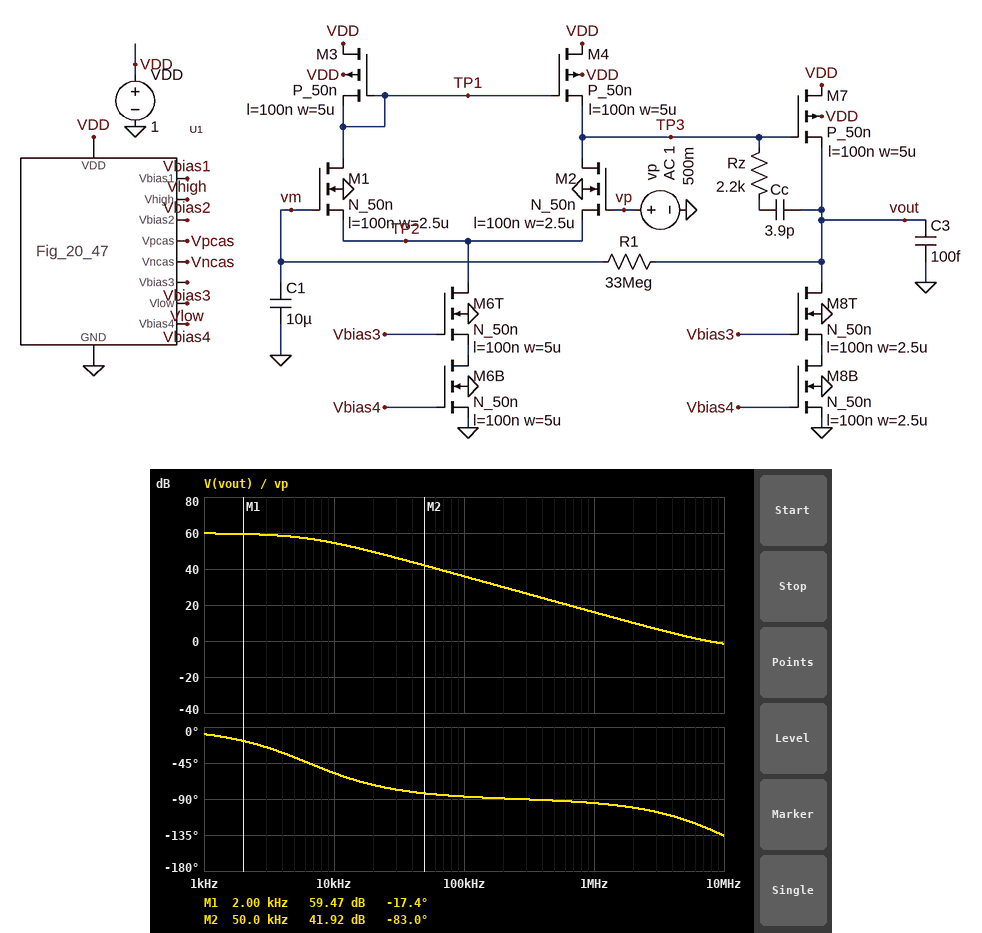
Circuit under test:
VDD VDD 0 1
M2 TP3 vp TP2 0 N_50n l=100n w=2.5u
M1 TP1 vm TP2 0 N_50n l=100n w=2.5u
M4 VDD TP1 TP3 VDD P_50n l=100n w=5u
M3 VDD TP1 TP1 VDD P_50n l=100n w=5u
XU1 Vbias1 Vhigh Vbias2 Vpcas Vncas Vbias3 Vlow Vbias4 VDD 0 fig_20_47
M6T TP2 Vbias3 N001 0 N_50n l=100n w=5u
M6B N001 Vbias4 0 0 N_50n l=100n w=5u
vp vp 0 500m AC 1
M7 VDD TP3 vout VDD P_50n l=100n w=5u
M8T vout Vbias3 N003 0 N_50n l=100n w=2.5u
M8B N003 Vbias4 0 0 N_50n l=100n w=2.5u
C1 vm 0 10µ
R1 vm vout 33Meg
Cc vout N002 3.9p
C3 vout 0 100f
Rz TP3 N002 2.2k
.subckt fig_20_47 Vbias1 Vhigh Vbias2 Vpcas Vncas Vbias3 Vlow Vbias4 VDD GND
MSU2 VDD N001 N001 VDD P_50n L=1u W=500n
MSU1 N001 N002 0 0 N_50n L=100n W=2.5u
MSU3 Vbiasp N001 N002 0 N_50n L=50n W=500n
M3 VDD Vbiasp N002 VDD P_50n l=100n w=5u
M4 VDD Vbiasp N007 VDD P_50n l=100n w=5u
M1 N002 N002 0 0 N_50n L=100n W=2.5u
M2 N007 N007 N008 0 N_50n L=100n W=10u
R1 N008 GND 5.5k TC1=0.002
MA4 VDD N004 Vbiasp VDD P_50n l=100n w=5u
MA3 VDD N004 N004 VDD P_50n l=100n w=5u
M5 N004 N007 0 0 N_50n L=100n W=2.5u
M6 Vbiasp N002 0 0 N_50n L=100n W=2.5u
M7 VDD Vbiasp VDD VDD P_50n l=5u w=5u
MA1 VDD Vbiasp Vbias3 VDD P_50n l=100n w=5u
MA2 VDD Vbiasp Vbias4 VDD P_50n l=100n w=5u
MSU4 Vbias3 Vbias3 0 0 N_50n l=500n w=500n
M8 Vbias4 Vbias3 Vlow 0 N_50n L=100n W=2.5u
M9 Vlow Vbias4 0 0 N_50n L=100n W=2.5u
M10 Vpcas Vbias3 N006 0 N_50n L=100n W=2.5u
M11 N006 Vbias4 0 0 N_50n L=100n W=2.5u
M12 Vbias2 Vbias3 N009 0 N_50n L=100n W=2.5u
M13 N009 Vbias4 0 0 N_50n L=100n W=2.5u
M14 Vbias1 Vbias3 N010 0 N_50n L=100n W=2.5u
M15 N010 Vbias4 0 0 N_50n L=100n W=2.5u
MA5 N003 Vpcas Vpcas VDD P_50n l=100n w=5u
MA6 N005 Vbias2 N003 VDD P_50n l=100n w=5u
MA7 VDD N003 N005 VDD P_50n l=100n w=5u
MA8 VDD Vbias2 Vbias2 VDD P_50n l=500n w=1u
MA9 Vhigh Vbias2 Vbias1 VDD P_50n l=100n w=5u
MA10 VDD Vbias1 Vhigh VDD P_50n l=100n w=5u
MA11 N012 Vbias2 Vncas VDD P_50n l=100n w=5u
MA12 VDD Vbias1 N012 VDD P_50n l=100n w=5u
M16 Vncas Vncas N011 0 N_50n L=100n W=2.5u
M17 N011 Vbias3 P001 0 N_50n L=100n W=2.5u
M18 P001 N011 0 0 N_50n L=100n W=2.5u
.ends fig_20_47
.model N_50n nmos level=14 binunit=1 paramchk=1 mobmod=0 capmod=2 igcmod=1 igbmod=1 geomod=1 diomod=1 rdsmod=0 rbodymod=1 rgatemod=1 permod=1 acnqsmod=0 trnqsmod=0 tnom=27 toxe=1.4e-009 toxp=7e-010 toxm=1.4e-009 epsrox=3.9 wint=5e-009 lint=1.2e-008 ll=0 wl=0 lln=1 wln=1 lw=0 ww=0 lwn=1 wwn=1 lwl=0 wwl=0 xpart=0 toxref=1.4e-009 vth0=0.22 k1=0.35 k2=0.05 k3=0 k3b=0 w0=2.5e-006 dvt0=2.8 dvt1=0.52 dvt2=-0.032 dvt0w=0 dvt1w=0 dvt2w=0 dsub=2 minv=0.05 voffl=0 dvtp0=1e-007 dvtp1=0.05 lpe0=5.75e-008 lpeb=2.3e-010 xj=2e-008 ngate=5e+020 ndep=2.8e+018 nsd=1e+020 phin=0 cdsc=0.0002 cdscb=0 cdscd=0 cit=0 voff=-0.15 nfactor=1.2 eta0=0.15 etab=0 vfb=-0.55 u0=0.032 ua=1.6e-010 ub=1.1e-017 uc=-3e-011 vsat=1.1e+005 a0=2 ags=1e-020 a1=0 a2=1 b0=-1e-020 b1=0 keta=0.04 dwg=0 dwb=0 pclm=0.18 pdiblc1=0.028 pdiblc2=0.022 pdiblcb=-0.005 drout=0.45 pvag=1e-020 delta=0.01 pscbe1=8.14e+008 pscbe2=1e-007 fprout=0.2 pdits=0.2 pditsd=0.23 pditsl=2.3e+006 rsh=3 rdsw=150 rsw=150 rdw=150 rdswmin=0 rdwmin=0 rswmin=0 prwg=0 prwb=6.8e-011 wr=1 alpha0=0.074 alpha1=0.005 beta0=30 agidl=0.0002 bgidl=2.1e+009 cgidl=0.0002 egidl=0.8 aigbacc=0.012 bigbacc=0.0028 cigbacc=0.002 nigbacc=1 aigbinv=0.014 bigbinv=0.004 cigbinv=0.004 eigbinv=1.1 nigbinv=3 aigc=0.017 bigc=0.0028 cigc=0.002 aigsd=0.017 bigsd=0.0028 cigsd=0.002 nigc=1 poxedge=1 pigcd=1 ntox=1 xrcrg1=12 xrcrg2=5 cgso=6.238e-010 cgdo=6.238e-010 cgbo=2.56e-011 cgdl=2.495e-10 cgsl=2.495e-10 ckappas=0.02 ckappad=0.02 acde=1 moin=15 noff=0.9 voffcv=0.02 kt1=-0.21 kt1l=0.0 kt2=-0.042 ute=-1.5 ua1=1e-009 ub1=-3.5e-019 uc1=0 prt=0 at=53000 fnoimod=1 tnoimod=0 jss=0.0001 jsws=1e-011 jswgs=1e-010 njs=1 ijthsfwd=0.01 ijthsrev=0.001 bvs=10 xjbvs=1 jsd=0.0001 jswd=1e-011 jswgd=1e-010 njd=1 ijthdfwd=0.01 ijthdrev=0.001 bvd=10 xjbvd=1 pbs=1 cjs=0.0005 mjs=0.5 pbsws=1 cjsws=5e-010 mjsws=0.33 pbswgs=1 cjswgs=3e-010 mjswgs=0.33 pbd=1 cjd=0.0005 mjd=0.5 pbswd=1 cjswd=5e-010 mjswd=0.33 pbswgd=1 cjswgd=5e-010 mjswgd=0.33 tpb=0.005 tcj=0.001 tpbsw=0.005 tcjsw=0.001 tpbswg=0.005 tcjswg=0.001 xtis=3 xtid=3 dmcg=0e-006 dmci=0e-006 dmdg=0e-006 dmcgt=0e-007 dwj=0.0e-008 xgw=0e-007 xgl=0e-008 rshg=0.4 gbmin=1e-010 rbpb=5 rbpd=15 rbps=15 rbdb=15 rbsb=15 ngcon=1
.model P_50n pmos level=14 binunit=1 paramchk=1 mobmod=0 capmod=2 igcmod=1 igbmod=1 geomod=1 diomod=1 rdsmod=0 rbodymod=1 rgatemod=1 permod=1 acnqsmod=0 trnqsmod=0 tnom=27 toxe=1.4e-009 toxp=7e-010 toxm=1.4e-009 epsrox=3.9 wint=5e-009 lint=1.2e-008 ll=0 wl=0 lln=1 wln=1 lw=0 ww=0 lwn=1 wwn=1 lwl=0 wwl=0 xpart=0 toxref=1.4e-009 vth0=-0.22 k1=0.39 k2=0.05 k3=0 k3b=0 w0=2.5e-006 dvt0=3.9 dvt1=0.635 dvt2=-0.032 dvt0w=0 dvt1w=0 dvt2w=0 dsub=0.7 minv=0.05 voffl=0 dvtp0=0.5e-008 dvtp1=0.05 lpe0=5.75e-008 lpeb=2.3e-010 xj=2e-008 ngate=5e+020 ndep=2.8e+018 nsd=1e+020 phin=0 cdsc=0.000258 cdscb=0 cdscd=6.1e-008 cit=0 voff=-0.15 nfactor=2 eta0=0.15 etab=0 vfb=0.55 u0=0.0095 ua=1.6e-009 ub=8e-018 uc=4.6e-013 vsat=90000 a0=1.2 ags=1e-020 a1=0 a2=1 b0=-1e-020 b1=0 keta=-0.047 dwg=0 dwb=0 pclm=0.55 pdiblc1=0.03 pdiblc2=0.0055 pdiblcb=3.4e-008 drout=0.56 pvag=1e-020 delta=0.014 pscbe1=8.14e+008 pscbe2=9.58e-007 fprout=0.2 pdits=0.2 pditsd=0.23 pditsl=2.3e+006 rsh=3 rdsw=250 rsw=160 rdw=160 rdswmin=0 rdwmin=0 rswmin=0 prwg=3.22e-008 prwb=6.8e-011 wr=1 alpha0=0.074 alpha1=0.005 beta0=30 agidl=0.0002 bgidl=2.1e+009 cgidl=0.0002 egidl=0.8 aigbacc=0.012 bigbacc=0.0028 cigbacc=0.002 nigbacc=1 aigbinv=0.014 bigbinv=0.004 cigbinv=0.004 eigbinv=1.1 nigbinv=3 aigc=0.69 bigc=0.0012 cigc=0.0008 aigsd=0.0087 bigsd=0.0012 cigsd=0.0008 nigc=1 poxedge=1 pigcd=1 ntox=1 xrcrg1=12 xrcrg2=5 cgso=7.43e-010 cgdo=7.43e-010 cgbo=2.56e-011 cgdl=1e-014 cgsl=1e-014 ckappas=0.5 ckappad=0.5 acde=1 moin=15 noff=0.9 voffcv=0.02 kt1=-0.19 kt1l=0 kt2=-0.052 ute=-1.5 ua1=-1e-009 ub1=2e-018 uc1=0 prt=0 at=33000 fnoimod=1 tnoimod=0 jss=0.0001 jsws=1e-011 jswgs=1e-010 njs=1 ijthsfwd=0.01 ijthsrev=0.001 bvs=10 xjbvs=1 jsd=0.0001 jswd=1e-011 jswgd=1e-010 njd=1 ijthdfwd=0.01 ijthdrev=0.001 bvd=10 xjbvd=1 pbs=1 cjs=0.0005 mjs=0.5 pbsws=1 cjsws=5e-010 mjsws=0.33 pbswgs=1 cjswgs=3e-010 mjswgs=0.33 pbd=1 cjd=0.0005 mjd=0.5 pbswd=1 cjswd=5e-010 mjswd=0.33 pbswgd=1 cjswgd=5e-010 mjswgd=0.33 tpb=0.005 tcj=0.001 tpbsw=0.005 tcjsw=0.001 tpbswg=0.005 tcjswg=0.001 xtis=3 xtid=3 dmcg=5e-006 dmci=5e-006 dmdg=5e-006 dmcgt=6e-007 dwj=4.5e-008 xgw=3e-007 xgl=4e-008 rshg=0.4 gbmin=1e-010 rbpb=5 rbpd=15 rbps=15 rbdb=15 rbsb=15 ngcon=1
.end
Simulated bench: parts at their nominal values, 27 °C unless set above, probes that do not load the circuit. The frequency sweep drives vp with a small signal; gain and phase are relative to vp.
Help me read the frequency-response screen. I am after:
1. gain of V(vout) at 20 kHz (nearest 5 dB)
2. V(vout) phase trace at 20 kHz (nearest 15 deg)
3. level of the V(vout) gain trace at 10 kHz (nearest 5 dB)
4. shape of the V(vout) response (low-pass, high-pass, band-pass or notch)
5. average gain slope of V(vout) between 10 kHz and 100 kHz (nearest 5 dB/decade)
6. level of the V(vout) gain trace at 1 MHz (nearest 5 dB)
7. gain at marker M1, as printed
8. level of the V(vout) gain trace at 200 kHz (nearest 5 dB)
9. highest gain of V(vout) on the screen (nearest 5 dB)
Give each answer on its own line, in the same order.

50 dB
-75 deg
55 dB
low-pass
-20 dB/decade
15 dB
59.47 dB
30 dB
60 dB
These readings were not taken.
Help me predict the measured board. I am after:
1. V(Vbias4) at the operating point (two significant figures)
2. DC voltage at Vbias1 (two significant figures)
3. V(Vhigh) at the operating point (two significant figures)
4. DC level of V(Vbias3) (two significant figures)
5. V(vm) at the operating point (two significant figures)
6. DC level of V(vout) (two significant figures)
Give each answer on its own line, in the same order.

360 mV
640 mV
790 mV
540 mV
500 mV
510 mV
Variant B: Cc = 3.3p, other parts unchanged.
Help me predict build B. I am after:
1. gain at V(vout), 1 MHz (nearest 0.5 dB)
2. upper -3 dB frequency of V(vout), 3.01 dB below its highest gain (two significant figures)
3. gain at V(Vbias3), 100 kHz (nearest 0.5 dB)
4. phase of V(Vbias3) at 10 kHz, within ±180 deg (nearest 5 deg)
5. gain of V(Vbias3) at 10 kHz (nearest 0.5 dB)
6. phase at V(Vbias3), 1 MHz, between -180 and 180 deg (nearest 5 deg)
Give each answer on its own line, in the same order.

17.5 dB
7.5 kHz
-52.5 dB
15 deg
-53.5 dB
10 deg
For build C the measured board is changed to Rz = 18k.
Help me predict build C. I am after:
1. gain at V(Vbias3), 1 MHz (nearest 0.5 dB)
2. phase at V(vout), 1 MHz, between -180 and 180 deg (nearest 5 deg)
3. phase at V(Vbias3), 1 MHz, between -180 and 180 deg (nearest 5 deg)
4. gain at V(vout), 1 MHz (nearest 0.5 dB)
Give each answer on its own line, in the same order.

-52.5 dB
-75 deg
30 deg
16.5 dB
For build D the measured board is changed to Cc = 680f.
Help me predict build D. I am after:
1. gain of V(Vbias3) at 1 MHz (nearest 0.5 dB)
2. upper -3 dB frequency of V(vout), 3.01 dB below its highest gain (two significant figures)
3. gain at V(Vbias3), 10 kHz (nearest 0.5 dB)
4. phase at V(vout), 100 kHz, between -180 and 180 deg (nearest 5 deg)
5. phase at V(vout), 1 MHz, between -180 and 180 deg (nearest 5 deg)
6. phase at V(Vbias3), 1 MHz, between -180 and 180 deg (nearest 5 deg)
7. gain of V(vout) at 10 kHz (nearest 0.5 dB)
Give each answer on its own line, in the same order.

-39.0 dB
36 kHz
-49.5 dB
-70 deg
-90 deg
5 deg
59.5 dB
